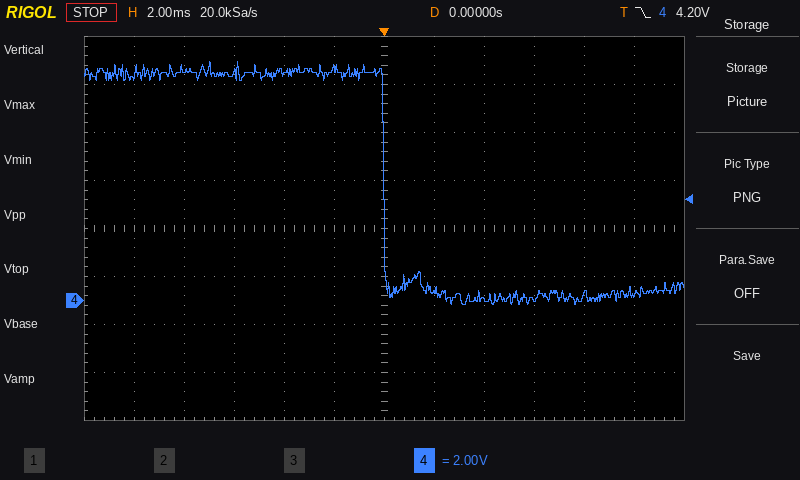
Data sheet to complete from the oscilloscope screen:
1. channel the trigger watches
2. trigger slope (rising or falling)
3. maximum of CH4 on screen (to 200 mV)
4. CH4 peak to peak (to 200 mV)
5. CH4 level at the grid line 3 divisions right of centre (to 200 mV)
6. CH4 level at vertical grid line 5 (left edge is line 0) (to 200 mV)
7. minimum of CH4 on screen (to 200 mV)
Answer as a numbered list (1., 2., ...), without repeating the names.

1. CH4
2. falling
3. 10.0 V
4. 10.2 V
5. 0.0 V
6. 9.6 V
7. -200 mV
